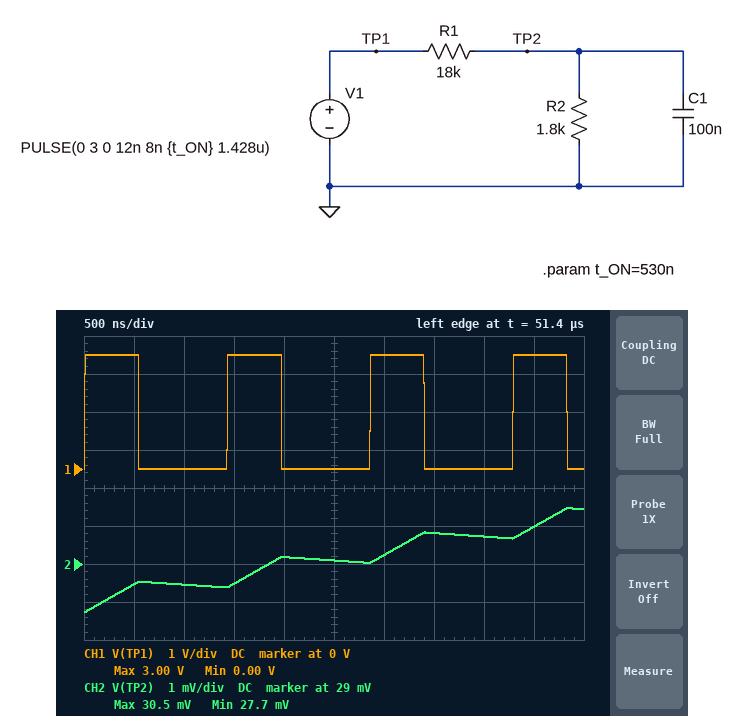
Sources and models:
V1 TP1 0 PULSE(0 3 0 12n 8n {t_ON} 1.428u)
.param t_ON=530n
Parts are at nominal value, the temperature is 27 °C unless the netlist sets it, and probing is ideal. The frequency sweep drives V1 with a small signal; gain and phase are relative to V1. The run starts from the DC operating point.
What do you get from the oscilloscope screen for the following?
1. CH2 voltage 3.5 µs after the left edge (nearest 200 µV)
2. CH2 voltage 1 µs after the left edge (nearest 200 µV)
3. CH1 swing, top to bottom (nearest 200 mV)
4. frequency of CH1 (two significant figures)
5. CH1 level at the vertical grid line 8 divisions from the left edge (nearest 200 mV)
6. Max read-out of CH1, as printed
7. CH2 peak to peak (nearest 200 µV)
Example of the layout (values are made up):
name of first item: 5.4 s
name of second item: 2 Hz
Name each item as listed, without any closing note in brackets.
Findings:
CH2 voltage 3.5 µs after the left edge: 29.8 mV
CH2 voltage 1 µs after the left edge: 28.4 mV
CH1 swing, top to bottom: 3.0 V
frequency of CH1: 700 kHz
CH1 level at the vertical grid line 8 divisions from the left edge: 0 V
Max read-out of CH1, as printed: 3.00 V
CH2 peak to peak: 2.8 mV
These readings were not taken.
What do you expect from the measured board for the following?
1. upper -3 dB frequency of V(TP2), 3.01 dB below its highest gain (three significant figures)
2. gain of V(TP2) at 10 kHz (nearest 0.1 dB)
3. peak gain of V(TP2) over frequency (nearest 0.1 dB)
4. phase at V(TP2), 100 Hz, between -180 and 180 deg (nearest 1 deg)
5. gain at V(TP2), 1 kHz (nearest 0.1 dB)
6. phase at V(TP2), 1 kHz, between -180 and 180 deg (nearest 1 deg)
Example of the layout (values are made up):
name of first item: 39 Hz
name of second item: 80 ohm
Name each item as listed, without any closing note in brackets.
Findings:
upper -3 dB frequency of V(TP2), 3.01 dB below its highest gain: 973 Hz
gain of V(TP2) at 10 kHz: -41.1 dB
peak gain of V(TP2) over frequency: -20.8 dB
phase at V(TP2), 100 Hz, between -180 and 180 deg: -6 deg
gain at V(TP2), 1 kHz: -24.0 dB
phase at V(TP2), 1 kHz, between -180 and 180 deg: -46 deg
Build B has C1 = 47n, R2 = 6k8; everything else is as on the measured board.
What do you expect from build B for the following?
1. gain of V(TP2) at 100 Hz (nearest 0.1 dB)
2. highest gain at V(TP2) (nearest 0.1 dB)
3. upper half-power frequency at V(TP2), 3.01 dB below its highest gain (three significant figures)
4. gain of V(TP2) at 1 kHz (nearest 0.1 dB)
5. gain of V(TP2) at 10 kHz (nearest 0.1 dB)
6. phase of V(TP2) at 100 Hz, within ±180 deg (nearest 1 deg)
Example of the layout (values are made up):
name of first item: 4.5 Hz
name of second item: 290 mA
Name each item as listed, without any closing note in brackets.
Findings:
gain of V(TP2) at 100 Hz: -11.3 dB
highest gain at V(TP2): -11.2 dB
upper half-power frequency at V(TP2), 3.01 dB below its highest gain: 686 Hz
gain of V(TP2) at 1 kHz: -16.2 dB
gain of V(TP2) at 10 kHz: -34.5 dB
phase of V(TP2) at 100 Hz, within ±180 deg: -8 deg
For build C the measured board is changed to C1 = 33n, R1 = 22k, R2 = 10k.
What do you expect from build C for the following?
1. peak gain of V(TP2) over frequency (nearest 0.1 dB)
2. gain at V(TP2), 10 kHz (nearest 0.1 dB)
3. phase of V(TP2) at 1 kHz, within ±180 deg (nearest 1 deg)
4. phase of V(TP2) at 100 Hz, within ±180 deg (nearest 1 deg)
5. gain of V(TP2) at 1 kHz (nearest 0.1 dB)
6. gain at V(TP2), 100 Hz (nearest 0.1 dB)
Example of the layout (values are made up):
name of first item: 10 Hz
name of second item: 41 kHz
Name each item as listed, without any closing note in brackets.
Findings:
peak gain of V(TP2) over frequency: -10.1 dB
gain at V(TP2), 10 kHz: -33.2 dB
phase of V(TP2) at 1 kHz, within ±180 deg: -55 deg
phase of V(TP2) at 100 Hz, within ±180 deg: -8 deg
gain of V(TP2) at 1 kHz: -14.9 dB
gain at V(TP2), 100 Hz: -10.2 dB
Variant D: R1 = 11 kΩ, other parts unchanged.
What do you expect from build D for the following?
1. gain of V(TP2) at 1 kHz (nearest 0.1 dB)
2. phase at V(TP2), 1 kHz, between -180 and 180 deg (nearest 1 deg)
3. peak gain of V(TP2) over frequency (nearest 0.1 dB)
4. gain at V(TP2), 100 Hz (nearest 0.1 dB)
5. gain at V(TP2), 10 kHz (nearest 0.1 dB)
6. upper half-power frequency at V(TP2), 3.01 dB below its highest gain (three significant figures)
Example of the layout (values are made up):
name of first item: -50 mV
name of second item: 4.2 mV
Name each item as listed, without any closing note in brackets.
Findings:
gain of V(TP2) at 1 kHz: -19.9 dB
phase at V(TP2), 1 kHz, between -180 and 180 deg: -44 deg
peak gain of V(TP2) over frequency: -17.0 dB
gain at V(TP2), 100 Hz: -17.1 dB
gain at V(TP2), 10 kHz: -36.8 dB
upper half-power frequency at V(TP2), 3.01 dB below its highest gain: 1.03 kHz
